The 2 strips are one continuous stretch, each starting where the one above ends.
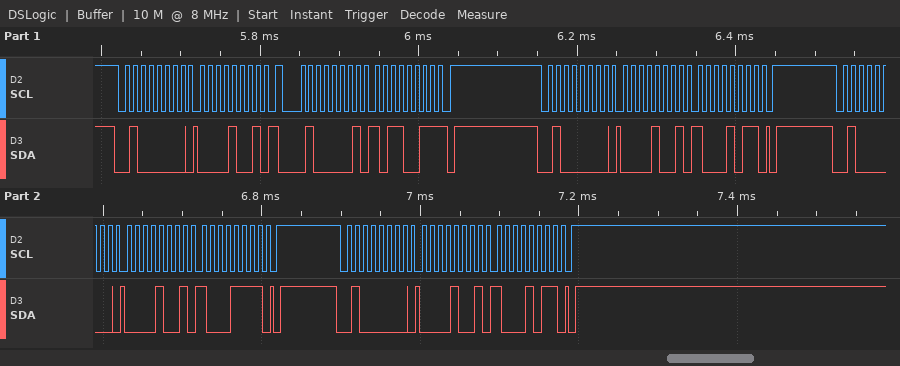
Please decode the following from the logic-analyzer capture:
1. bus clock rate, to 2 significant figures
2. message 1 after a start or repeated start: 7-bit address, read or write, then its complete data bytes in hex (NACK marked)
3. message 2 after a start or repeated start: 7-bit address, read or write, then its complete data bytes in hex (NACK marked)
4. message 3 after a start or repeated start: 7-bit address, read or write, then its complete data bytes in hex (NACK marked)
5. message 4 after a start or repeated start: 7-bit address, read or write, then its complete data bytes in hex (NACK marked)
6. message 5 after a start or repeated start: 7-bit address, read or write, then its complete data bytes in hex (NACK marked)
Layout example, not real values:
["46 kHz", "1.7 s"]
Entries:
["100 kHz", "0x20 write: 09", "0x20 read: B3 NACK", "0x20 write: 09 8B", "0x20 write: 09 8F", "0x20 write: 09 8B"]
